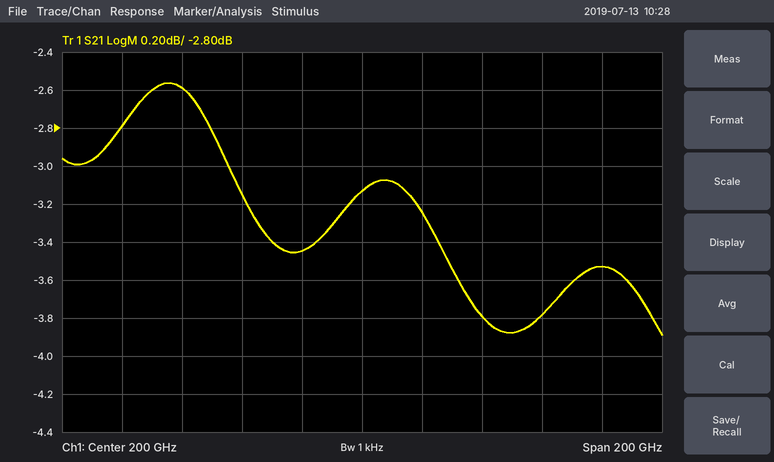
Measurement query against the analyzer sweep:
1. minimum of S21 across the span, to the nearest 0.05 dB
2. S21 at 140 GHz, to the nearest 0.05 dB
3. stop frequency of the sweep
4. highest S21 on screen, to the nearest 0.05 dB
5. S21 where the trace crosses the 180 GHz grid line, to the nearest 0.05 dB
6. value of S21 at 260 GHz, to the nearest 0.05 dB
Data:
-3.90 dB
-2.60 dB
300 GHz
-2.55 dB
-3.45 dB
-3.80 dB
